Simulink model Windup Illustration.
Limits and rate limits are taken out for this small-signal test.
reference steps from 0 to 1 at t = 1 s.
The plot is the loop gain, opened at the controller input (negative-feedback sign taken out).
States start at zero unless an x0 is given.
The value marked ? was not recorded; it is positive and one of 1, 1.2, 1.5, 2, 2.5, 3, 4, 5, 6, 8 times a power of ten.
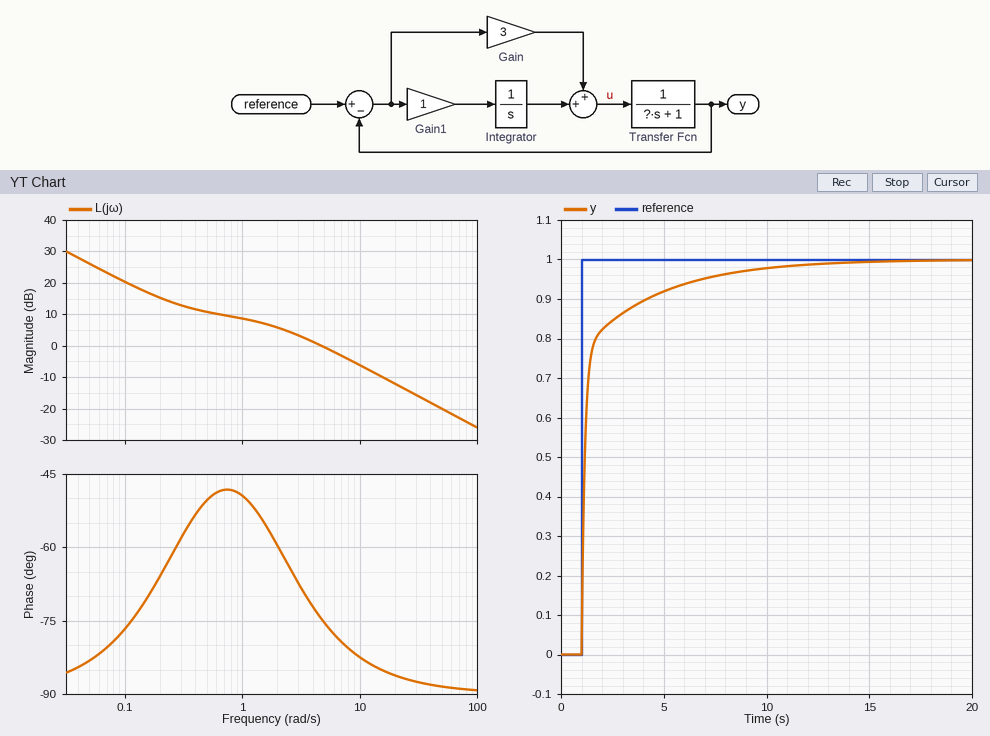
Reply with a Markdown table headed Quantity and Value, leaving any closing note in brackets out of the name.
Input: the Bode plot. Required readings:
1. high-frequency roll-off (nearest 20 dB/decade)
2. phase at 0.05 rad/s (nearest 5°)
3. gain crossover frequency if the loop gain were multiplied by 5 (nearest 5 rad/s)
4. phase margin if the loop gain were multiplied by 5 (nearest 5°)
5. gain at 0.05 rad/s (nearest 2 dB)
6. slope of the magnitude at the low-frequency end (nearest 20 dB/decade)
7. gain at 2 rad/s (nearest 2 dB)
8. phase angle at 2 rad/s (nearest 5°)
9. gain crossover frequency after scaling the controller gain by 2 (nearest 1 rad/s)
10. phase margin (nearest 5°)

| Quantity | Value |
|---|---|
| high-frequency roll-off | -20 dB/decade |
| phase at 0.05 rad/s | -85° |
| gain crossover frequency if the loop gain were multiplied by 5 | 25 rad/s |
| phase margin if the loop gain were multiplied by 5 | 95° |
| gain at 0.05 rad/s | 26 dB |
| slope of the magnitude at the low-frequency end | -20 dB/decade |
| gain at 2 rad/s | 6 dB |
| phase angle at 2 rad/s | -60° |
| gain crossover frequency after scaling the controller gain by 2 | 10 rad/s |
| phase margin | 105° |
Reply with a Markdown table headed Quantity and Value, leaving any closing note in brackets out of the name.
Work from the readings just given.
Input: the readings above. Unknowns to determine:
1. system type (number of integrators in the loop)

| Quantity | Value |
|---|---|
| system type | 1 |
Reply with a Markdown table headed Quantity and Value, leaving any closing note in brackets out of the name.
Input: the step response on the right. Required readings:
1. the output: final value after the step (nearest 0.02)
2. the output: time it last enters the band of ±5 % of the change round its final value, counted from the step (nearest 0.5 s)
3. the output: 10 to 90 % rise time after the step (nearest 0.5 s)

| Quantity | Value |
|---|---|
| the output: final value after the step | 1.00 |
| the output: time it last enters the band of ±5 % of the change round its final value, counted from the step | 6.0 s |
| the output: 10 to 90 % rise time after the step | 3.0 s |
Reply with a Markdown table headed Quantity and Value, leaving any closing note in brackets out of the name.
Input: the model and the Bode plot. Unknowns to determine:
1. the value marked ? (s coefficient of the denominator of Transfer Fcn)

| Quantity | Value |
|---|---|
| the value marked ? | 0.6 |
